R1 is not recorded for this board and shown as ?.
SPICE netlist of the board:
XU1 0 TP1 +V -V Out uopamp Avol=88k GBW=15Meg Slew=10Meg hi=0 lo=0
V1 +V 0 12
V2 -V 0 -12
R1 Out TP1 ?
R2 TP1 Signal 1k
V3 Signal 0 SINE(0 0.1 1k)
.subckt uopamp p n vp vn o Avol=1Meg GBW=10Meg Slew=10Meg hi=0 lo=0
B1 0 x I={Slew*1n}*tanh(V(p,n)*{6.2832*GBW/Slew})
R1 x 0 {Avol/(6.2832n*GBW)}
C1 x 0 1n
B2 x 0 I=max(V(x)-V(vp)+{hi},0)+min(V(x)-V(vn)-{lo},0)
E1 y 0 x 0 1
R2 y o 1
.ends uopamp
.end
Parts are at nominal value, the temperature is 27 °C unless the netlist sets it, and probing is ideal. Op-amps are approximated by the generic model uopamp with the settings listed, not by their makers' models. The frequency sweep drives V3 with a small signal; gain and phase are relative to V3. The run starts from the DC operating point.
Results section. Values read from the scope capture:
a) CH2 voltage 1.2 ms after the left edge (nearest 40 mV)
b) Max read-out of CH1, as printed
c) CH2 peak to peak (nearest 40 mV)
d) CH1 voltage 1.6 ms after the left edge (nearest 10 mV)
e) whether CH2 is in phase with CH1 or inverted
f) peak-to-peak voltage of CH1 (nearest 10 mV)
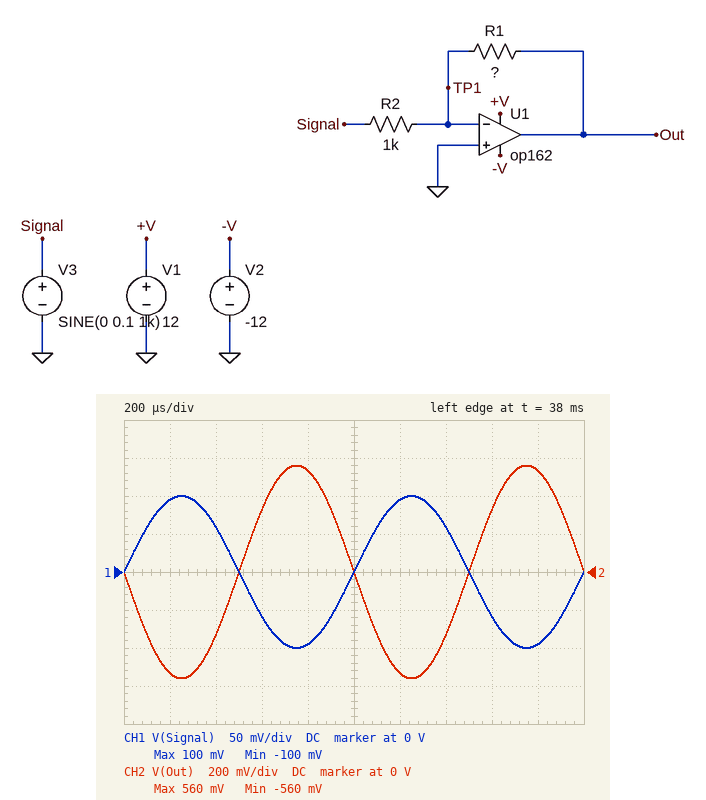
-520 mV
100 mV
1.12 V
-60 mV
inverted
200 mV
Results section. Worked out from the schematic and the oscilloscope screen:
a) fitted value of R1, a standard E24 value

5.6 kΩ
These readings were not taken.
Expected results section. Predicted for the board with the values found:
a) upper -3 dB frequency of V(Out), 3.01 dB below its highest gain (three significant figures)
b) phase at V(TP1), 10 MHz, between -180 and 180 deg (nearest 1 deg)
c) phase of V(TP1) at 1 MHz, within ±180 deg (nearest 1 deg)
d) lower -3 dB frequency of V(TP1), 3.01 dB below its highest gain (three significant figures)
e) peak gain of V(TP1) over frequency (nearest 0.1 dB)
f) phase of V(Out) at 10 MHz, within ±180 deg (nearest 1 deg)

2.27 MHz
13 deg
66 deg
2.27 MHz
-1.4 dB
103 deg
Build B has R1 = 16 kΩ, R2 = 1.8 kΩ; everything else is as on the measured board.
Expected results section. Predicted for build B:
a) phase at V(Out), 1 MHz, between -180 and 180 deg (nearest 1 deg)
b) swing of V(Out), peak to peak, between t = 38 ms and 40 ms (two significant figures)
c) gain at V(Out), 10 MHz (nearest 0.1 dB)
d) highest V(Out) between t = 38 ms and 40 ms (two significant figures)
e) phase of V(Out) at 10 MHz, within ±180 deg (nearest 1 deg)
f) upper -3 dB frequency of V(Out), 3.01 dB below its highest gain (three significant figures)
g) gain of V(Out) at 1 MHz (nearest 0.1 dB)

147 deg
1.8 V
2.5 dB
890 mV
99 deg
1.52 MHz
17.4 dB
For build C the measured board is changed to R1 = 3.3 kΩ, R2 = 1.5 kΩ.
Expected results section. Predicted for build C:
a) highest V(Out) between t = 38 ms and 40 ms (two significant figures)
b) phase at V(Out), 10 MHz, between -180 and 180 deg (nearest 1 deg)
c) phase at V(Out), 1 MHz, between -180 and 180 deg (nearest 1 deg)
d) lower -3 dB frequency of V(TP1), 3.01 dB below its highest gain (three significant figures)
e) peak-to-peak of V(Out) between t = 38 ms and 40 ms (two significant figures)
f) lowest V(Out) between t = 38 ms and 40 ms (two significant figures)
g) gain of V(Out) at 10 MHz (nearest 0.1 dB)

220 mV
115 deg
168 deg
4.69 MHz
440 mV
-220 mV
-0.6 dB
